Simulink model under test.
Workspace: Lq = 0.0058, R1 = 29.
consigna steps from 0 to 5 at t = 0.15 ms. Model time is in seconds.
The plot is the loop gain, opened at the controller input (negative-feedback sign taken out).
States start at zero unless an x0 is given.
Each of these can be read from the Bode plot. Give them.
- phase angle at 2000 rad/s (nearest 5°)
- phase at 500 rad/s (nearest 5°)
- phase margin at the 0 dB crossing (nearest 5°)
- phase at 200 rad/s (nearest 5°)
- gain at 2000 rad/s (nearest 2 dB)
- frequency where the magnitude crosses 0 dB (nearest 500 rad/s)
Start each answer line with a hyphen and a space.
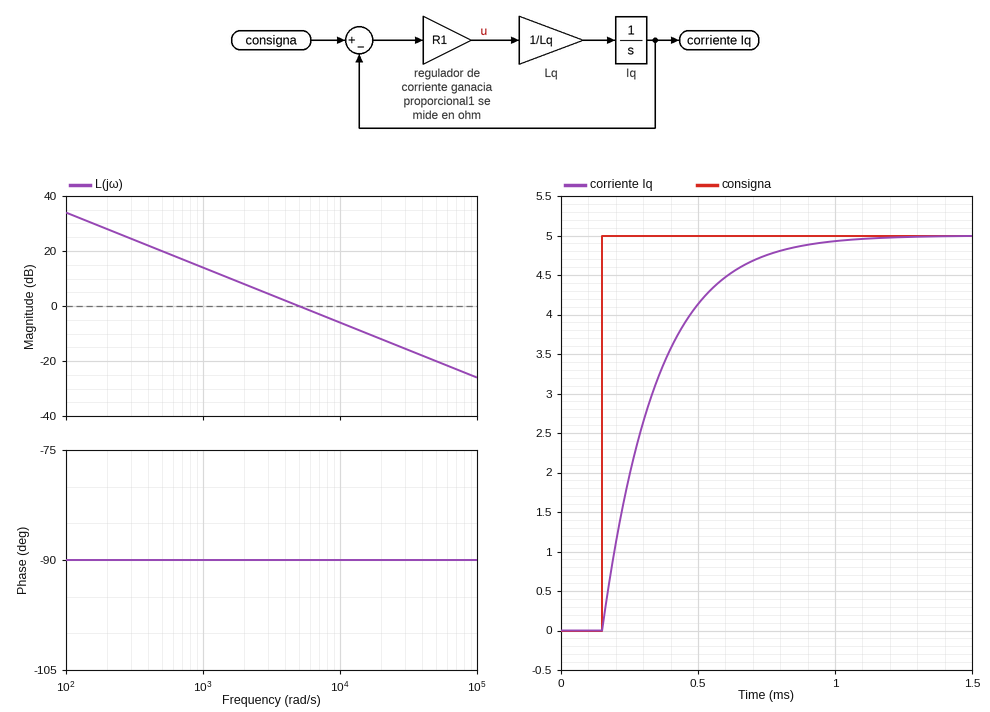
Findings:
- -90°
- -90°
- 90°
- -90°
- 8 dB
- 5000 rad/s
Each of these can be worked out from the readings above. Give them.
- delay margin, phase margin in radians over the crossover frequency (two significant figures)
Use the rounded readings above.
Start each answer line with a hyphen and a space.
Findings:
- 0.00031 s
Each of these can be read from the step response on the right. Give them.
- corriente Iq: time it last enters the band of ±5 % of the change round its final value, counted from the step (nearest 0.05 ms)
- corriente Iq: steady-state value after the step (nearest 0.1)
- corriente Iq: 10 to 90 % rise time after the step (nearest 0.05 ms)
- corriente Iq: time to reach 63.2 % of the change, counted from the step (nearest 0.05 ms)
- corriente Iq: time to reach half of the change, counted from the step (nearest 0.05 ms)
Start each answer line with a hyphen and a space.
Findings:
- 0.60 ms
- 5.0
- 0.45 ms
- 0.20 ms
- 0.15 ms
